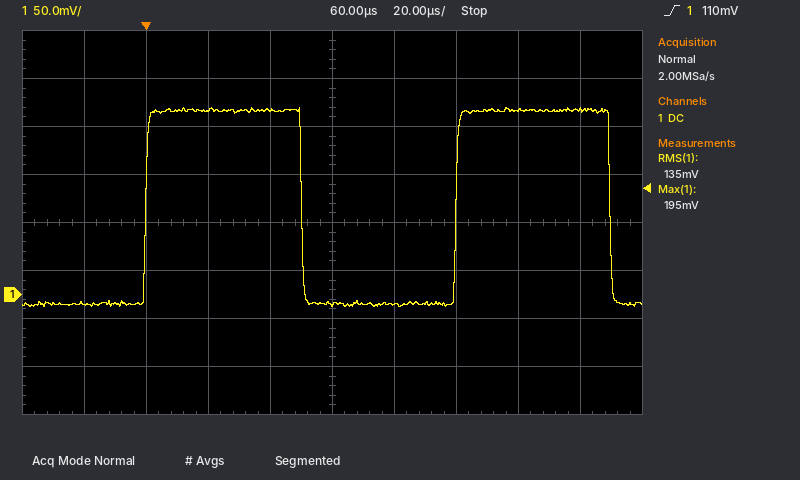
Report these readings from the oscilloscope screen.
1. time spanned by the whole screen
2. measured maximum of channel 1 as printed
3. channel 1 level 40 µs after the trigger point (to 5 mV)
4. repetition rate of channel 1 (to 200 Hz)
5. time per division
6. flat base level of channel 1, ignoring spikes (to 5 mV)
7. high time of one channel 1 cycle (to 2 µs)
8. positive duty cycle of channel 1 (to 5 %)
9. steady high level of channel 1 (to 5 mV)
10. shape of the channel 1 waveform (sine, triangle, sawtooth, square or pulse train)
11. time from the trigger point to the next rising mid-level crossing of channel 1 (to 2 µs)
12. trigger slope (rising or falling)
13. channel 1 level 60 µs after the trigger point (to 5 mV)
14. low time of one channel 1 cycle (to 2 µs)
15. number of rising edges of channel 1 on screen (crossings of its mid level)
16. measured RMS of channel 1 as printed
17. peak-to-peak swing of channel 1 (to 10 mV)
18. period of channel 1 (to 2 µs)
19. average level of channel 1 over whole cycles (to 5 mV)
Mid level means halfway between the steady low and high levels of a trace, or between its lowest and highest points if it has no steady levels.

200 µs
195 mV
190 mV
10.0 kHz
20 µs
-10 mV
50 µs
50 %
190 mV
square
100 µs
rising
-10 mV
50 µs
2
135 mV
210 mV
100 µs
90 mV
